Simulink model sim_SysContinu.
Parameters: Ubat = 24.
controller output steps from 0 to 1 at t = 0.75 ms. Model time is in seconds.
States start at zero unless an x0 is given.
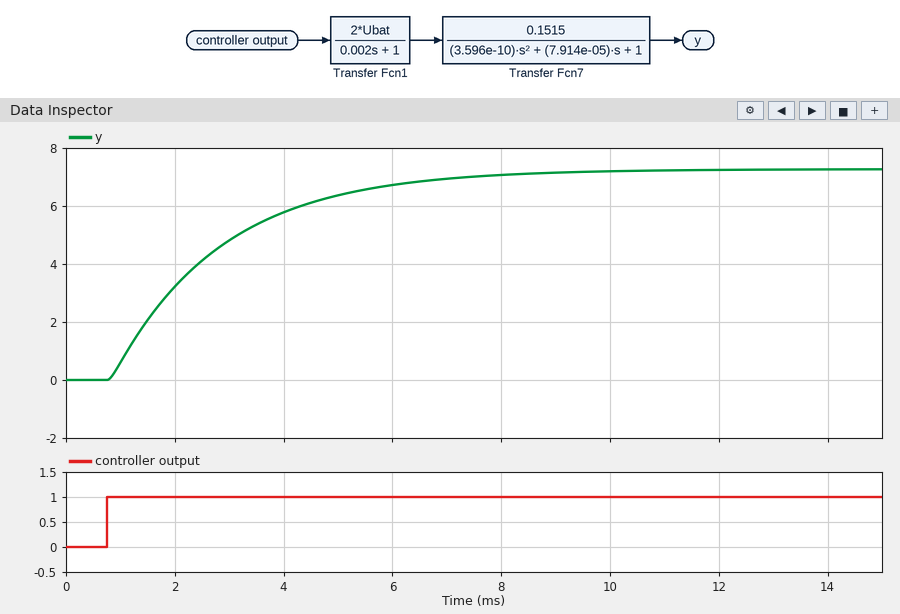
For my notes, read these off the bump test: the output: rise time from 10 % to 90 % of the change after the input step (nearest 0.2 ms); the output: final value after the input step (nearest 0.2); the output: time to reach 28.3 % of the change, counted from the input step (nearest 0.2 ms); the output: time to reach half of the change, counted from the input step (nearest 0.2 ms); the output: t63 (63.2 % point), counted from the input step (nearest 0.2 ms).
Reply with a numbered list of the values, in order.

1. 4.4 ms
2. 7.2
3. 0.8 ms
4. 1.4 ms
5. 2.0 ms
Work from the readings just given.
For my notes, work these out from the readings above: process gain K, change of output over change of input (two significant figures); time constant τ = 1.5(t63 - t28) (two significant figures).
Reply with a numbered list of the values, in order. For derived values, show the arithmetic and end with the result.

1. (7.2 - 0) / 1 = 7.2
2. 1.5 × (2 - 0.8) = 1.8 ms
